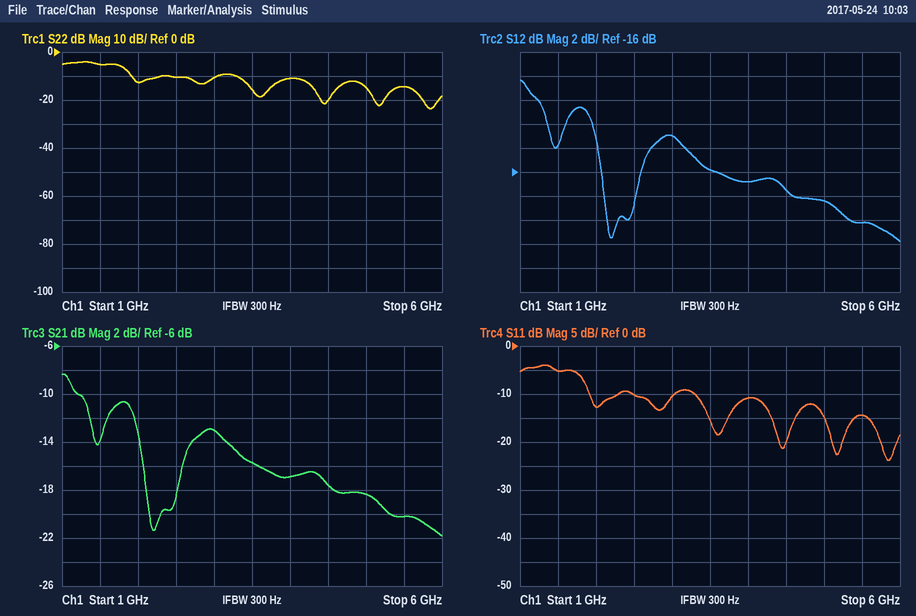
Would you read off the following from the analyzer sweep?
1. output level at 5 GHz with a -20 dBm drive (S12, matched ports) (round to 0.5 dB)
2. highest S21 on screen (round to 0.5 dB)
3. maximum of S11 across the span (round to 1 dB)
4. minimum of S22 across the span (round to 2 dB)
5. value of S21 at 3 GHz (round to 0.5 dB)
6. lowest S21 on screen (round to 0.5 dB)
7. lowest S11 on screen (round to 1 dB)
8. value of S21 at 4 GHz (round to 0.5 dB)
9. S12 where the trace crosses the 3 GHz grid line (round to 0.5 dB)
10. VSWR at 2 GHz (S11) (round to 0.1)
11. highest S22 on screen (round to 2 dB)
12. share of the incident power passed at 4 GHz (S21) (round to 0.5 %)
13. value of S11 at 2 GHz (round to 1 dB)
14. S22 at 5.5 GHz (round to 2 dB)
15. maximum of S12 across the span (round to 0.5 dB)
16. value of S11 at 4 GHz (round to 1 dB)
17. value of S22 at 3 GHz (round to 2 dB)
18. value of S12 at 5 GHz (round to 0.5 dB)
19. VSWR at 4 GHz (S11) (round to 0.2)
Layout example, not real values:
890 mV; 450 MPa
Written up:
-38.5 dBm; -8.5 dB; -4 dB; -24 dB; -13.0 dB; -22.0 dB; -24 dB; -17.0 dB; -13.0 dB; 1.6; -4 dB; 2.0 %; -13 dB; -14 dB; -8.5 dB; -11 dB; -10 dB; -18.5 dB; 1.8
